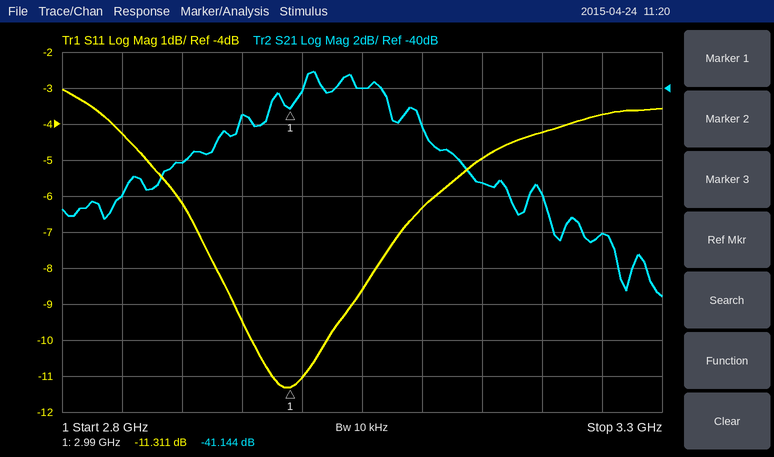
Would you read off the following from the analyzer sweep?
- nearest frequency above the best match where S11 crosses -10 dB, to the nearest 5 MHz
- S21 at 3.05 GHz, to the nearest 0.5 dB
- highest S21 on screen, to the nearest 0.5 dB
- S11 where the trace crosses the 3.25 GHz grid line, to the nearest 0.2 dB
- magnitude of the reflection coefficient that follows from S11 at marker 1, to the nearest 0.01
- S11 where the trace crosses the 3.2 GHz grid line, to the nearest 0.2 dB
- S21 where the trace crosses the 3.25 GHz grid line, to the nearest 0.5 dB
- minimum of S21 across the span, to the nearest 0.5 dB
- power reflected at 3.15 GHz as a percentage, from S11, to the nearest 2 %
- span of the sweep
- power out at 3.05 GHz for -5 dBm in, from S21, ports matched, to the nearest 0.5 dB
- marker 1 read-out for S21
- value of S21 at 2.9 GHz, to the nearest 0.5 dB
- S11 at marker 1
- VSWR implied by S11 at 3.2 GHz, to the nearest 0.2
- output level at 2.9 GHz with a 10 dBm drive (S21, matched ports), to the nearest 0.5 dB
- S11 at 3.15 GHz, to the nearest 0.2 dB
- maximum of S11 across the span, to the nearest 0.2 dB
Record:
3.020 GHz
-40.0 dB
-39.0 dB
-3.8 dB
0.27
-4.2 dB
-48.0 dB
-51.5 dB
32 %
500 MHz
-45.0 dBm
-41.144 dB
-44.0 dB
-11.311 dB
4.2
-34.0 dBm
-5.0 dB
-3.0 dB
